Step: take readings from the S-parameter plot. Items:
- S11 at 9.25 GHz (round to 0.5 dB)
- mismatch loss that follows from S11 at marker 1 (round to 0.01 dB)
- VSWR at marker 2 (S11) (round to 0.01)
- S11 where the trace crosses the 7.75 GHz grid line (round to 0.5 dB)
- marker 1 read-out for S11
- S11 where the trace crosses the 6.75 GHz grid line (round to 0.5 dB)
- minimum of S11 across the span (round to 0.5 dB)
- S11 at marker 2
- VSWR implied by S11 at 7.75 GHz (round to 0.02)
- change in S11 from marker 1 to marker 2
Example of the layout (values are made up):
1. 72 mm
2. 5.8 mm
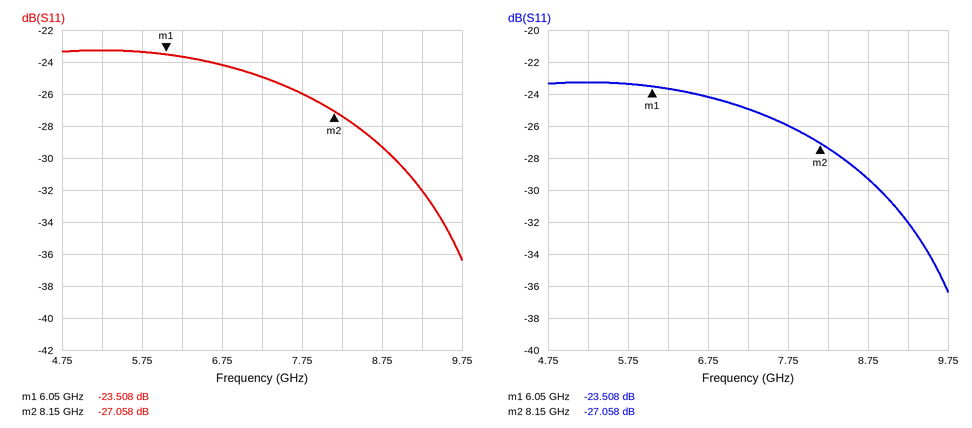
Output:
1. -32.0 dB
2. 0.02 dB
3. 1.09
4. -26.0 dB
5. -23.508 dB
6. -24.0 dB
7. -36.5 dB
8. -27.058 dB
9. 1.10
10. -3.550 dB
